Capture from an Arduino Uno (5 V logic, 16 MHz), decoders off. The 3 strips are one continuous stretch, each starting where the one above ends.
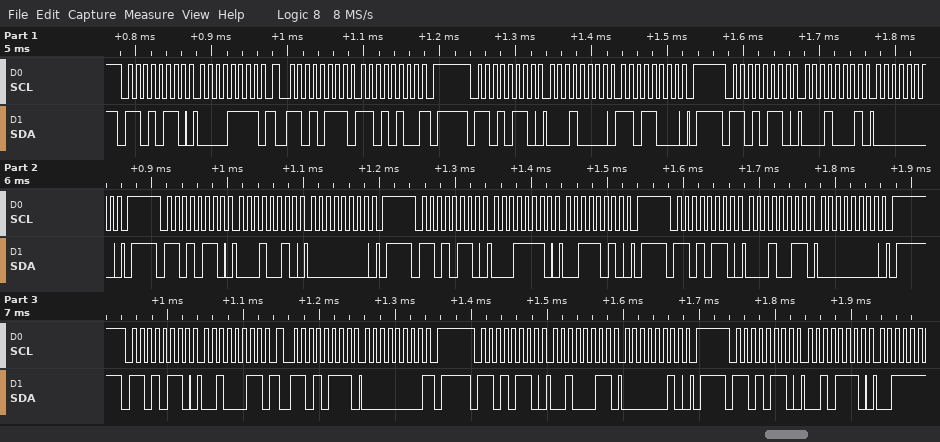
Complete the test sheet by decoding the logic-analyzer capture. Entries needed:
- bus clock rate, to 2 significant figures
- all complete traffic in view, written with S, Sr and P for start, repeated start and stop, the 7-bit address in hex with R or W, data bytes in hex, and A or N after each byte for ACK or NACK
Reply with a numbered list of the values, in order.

1. 100 kHz
2. S 6BW A 0F A Sr 6BR A D4 N P S 6BW A 10 A D8 A P S 6BW A 11 A 00 A P S 6BW A 12 A 00 A P S 6BW A 1E A 3A A P S 6BW A 13 A 00 A P S 6BW A 23 A Sr 6BR A 00 N P S 6BW A 23 A 02 A P S 6BW A 2E A
